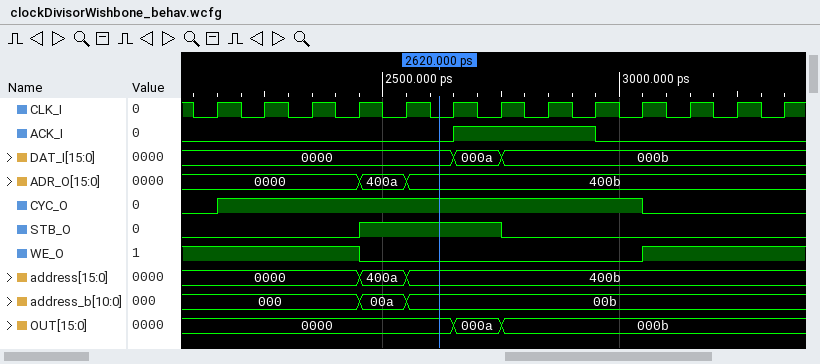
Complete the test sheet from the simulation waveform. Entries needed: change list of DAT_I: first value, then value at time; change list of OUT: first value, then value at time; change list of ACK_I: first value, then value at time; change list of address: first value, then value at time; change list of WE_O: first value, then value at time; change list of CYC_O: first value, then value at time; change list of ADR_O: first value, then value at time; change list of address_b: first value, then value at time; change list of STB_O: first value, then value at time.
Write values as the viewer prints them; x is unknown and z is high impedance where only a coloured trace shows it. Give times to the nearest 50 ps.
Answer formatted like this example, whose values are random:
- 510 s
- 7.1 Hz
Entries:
- 0000, 000a at 2650 ps, 000b at 2750 ps
- 0000, 000a at 2650 ps, 000b at 2750 ps
- 0, 1 at 2650 ps, 0 at 2950 ps
- 0000, 400a at 2450 ps, 400b at 2550 ps
- 1, 0 at 2450 ps, 1 at 3050 ps
- 0, 1 at 2150 ps, 0 at 3050 ps
- 0000, 400a at 2450 ps, 400b at 2550 ps
- 000, 00a at 2450 ps, 00b at 2550 ps
- 0, 1 at 2450 ps, 0 at 2750 ps
